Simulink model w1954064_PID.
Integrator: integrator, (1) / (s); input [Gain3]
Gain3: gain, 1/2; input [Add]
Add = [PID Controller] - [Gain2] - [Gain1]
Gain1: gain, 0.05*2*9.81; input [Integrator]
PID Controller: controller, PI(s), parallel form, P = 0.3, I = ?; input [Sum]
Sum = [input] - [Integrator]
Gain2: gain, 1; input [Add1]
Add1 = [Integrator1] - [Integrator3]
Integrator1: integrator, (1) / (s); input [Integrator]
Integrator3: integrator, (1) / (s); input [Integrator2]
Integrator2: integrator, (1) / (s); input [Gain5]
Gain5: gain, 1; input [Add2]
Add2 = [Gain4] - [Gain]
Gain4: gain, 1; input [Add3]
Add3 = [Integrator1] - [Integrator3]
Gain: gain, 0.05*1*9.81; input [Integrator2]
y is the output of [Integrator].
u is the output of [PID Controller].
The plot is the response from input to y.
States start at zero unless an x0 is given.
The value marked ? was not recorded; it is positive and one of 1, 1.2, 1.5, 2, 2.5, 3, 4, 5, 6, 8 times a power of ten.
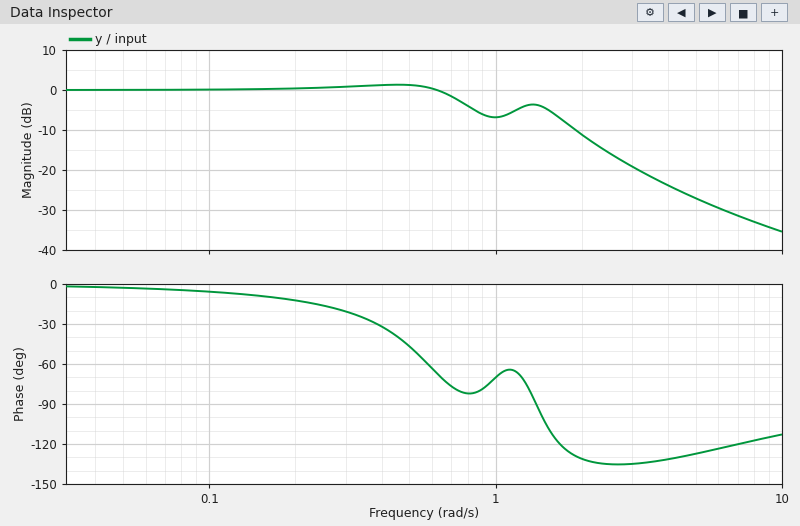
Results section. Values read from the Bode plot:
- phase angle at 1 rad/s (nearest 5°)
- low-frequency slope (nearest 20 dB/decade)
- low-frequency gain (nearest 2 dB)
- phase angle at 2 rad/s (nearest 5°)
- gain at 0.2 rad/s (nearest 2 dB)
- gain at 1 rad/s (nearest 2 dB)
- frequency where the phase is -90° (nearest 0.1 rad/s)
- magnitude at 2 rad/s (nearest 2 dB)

-70°
0 dB/decade
0 dB
-130°
0 dB
-6 dB
1.4 rad/s
-12 dB
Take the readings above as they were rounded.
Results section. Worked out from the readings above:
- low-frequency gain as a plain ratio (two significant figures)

1.0
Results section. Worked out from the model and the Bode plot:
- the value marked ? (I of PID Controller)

1.5
